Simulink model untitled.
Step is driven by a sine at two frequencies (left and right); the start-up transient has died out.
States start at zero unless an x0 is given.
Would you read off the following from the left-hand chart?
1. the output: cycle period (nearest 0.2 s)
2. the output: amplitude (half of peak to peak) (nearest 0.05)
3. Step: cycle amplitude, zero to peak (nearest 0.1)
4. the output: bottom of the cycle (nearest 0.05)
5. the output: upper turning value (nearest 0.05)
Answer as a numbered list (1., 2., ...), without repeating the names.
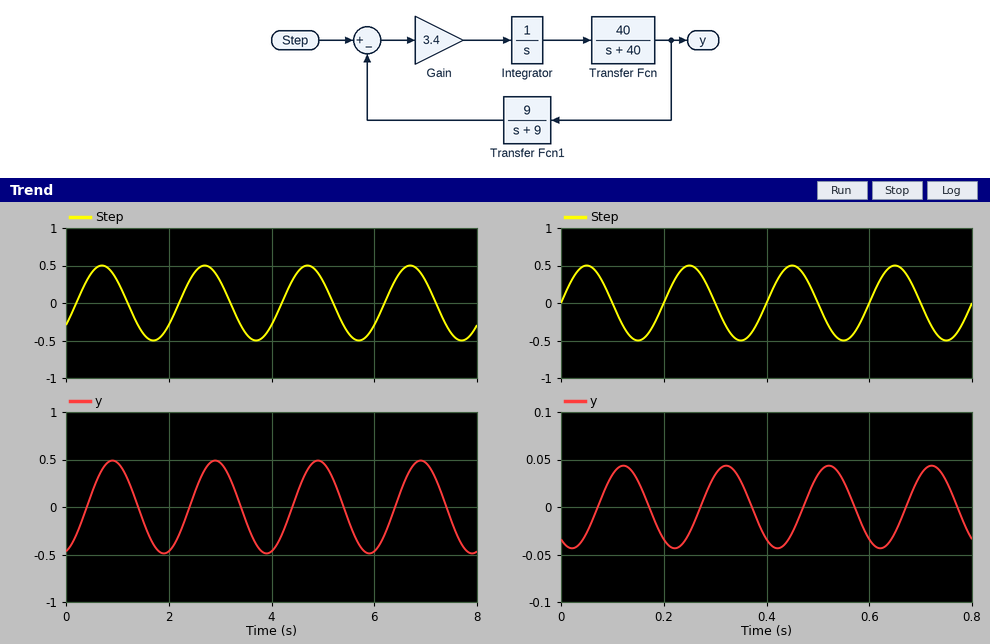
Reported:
1. 2.0 s
2. 0.50
3. 0.5
4. -0.50
5. 0.50
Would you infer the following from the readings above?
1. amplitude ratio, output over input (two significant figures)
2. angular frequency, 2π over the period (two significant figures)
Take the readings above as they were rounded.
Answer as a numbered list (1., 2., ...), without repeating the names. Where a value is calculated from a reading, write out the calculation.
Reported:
1. 0.5 / 0.5 = 1.0
2. 2π / 2 = 3.1 rad/s
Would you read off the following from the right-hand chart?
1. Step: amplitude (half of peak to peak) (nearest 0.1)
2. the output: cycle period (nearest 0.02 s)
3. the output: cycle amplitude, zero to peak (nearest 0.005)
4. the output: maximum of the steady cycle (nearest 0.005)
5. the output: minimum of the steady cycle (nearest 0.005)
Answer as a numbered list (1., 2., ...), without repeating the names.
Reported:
1. 0.5
2. 0.20 s
3. 0.045
4. 0.045
5. -0.045
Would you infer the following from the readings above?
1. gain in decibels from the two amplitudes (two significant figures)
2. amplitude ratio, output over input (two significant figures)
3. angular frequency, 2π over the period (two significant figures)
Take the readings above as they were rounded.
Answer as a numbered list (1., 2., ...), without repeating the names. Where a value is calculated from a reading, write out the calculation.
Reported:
1. 20 log10(0.045 / 0.5) = -21 dB
2. 0.045 / 0.5 = 0.090
3. 2π / 0.2 = 31 rad/s
